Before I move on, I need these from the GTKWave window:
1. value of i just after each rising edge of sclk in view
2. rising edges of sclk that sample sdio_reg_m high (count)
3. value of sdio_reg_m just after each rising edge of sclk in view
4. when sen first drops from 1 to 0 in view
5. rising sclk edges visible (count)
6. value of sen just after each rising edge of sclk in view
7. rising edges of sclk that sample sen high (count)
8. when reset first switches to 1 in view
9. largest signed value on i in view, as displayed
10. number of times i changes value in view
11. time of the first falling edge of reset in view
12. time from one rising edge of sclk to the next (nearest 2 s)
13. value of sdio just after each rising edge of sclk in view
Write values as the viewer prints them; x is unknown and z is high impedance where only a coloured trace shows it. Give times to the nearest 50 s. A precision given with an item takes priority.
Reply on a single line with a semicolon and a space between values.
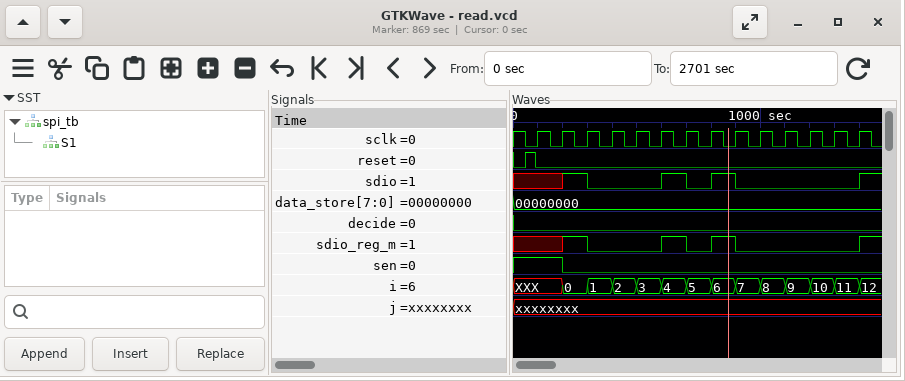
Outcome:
XXX, 0, 1, 2, 3, 4, 5, 6, 7, 8, 9, 10, 11, 12; 3; x 1 0 0 0 1 0 1 0 0 0 0 0 1; 200 s; 14; 1 0 0 0 0 0 0 0 0 0 0 0 0 0; 2; 50 s; 12; 13; 100 s; 100 s; x 1 0 0 0 1 0 1 0 0 0 0 0 1
